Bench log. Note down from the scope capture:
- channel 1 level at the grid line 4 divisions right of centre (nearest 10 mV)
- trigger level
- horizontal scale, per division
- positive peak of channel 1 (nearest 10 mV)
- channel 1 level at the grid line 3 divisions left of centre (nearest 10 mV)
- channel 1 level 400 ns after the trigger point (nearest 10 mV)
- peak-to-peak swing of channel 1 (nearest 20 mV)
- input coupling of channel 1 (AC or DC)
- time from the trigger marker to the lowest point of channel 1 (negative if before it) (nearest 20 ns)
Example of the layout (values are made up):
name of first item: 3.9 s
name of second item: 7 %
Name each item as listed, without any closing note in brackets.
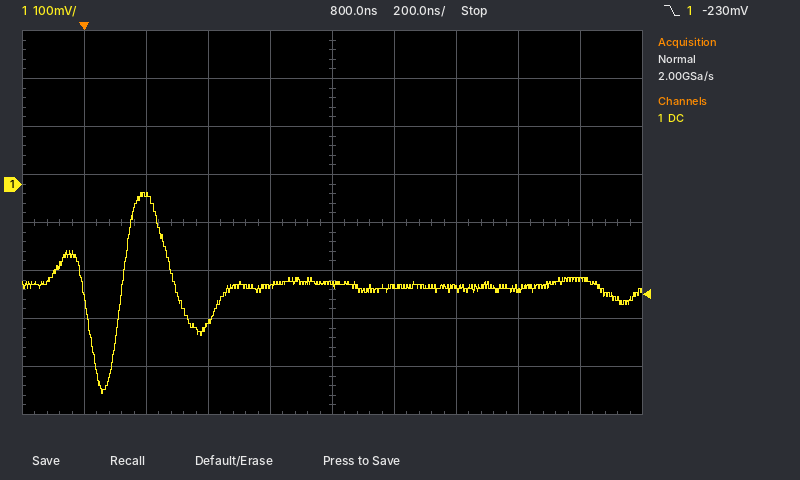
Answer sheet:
channel 1 level at the grid line 4 divisions right of centre: -200 mV
trigger level: -230 mV
horizontal scale, per division: 200 ns
positive peak of channel 1: -20 mV
channel 1 level at the grid line 3 divisions left of centre: -20 mV
channel 1 level 400 ns after the trigger point: -290 mV
peak-to-peak swing of channel 1: 420 mV
input coupling of channel 1: DC
time from the trigger marker to the lowest point of channel 1 (negative if before it): +60 ns
